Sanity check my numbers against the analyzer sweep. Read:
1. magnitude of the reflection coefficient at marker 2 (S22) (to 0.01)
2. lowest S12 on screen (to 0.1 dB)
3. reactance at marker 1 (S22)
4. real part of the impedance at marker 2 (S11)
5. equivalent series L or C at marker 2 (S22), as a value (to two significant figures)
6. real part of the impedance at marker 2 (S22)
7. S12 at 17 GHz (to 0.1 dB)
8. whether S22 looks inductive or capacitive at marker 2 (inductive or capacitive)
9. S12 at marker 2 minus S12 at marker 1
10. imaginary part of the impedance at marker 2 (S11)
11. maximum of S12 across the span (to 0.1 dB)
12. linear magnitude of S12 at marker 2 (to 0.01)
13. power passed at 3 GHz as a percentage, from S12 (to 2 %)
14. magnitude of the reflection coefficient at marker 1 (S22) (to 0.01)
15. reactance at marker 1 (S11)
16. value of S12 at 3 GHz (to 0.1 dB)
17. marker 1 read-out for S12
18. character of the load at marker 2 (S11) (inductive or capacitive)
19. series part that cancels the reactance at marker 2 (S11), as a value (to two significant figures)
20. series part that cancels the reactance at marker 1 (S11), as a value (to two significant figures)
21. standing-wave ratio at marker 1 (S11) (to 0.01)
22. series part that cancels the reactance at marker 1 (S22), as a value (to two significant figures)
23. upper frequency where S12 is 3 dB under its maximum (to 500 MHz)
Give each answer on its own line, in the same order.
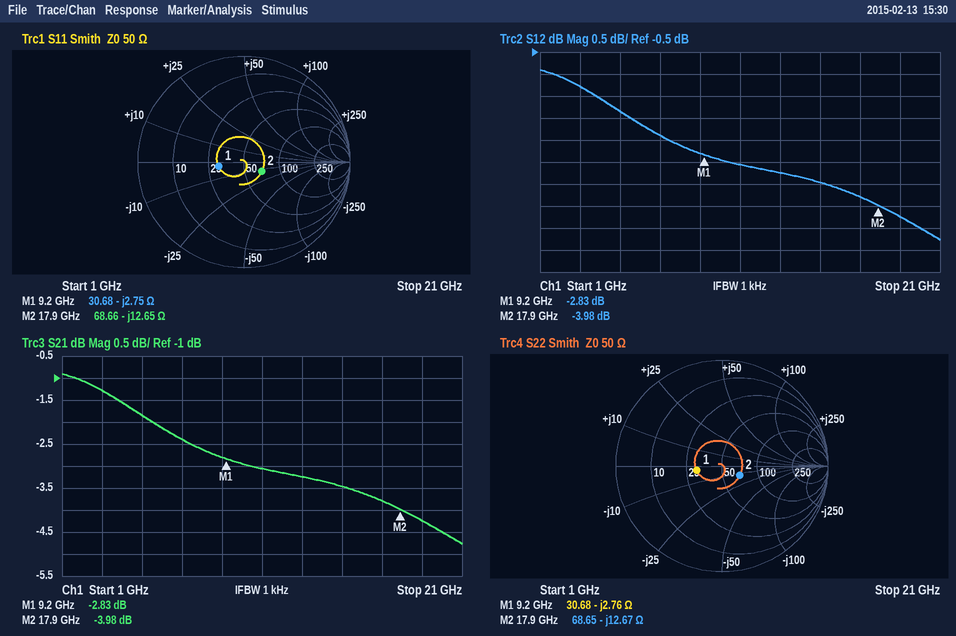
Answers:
0.19
-4.8 dB
-2.76 Ω
68.66 Ω
700 fF
68.65 Ω
-3.8 dB
capacitive
-1.15 dB
-12.65 Ω
-0.9 dB
0.63
74 %
0.24
-2.75 Ω
-1.3 dB
-2.83 dB
capacitive
110 pH
48 pH
1.64
48 pH
17.5 GHz
